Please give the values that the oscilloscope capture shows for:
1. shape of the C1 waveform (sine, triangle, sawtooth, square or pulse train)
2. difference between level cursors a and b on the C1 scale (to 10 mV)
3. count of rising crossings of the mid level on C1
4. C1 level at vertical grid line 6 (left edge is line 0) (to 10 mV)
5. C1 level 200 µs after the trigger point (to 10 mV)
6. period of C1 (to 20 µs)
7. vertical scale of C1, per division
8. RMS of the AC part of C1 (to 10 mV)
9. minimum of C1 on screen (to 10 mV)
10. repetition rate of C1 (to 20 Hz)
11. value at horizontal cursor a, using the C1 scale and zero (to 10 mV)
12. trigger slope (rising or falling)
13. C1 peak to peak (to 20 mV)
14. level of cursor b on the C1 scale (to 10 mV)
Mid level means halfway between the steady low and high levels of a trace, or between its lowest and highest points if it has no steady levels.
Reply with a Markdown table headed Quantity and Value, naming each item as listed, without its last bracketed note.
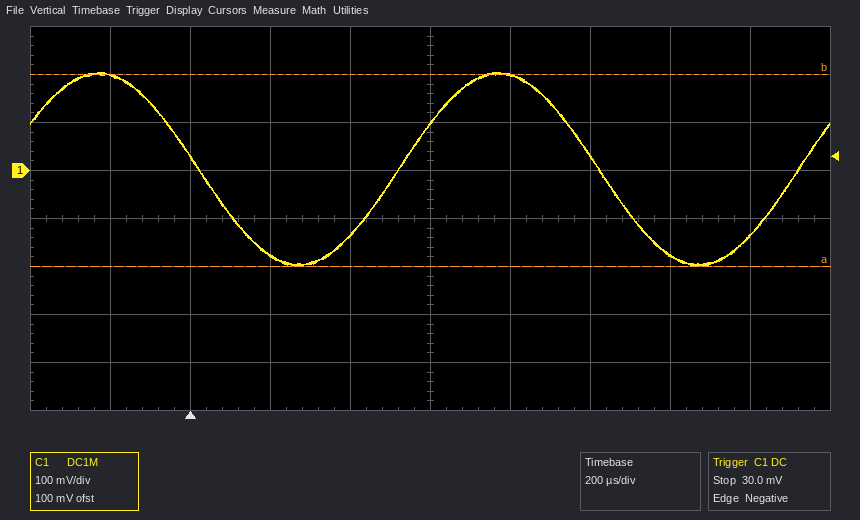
| Quantity | Value |
|---|---|
| shape of the C1 waveform | sine |
| difference between level cursors a and b on the C1 scale | 400 mV |
| count of rising crossings of the mid level on C1 | 2 |
| C1 level at vertical grid line 6 (left edge is line 0) | 200 mV |
| C1 level 200 µs after the trigger point | -180 mV |
| period of C1 | 1.00 ms |
| vertical scale of C1, per division | 100 mV |
| RMS of the AC part of C1 | 140 mV |
| minimum of C1 on screen | -200 mV |
| repetition rate of C1 | 1.00 kHz |
| value at horizontal cursor a, using the C1 scale and zero | -200 mV |
| trigger slope | falling |
| C1 peak to peak | 400 mV |
| level of cursor b on the C1 scale | 200 mV |
